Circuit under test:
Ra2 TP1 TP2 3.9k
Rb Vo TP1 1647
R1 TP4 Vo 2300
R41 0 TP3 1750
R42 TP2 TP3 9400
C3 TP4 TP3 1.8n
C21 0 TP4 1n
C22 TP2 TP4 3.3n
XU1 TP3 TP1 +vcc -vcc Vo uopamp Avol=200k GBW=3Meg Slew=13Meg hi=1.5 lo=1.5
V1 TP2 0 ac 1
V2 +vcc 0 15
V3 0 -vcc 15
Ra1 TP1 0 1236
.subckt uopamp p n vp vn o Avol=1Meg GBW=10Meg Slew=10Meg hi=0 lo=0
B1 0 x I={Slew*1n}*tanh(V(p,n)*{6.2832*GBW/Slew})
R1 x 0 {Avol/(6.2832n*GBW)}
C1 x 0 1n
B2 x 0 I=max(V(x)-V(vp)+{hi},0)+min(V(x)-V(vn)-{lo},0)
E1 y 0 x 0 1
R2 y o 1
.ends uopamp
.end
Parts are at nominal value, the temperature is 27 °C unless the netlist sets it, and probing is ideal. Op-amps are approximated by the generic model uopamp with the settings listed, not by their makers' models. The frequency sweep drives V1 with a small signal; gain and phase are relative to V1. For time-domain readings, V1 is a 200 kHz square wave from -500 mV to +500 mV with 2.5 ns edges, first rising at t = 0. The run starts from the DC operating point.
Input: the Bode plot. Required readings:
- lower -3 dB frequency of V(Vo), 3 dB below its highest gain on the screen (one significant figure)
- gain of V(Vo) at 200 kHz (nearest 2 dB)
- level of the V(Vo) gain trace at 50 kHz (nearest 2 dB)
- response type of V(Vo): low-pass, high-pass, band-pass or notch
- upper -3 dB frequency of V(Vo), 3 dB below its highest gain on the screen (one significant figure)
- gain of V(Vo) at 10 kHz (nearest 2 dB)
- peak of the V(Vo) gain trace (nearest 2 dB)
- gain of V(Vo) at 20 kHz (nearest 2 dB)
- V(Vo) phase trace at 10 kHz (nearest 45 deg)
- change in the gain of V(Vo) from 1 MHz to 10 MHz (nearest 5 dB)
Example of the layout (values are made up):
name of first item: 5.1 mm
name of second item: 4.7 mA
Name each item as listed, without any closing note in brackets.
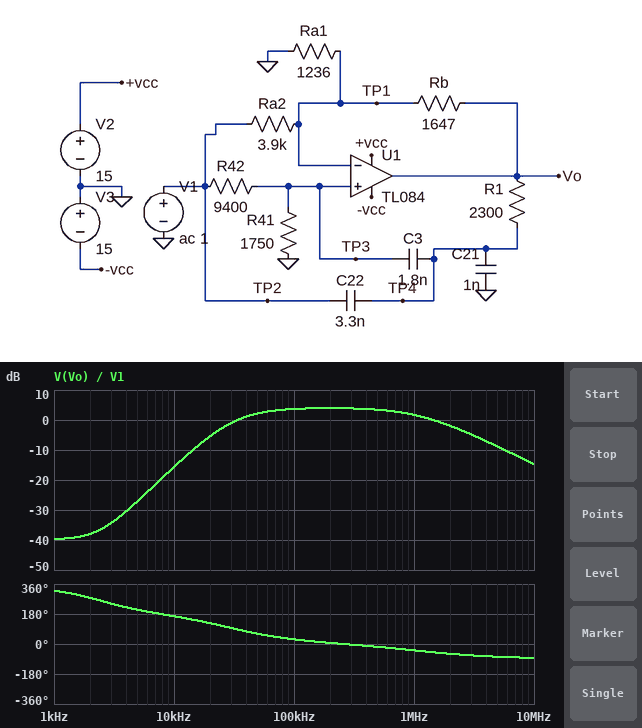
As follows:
lower -3 dB frequency of V(Vo), 3 dB below its highest gain on the screen: 40 kHz
gain of V(Vo) at 200 kHz: 4 dB
level of the V(Vo) gain trace at 50 kHz: 2 dB
response type of V(Vo): low-pass, high-pass, band-pass or notch: band-pass
upper -3 dB frequency of V(Vo), 3 dB below its highest gain on the screen: 1 MHz
gain of V(Vo) at 10 kHz: -16 dB
peak of the V(Vo) gain trace: 4 dB
gain of V(Vo) at 20 kHz: -6 dB
V(Vo) phase trace at 10 kHz: 180 deg
change in the gain of V(Vo) from 1 MHz to 10 MHz: -15 dB
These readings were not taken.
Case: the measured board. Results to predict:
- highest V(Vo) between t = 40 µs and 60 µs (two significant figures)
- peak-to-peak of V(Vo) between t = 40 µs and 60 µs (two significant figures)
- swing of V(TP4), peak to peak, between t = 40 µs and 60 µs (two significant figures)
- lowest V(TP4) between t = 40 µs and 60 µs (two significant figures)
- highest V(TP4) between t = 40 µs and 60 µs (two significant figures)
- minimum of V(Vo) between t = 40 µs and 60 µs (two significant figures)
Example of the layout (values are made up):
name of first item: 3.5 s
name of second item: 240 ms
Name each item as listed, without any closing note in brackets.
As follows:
highest V(Vo) between t = 40 µs and 60 µs: 980 mV
peak-to-peak of V(Vo) between t = 40 µs and 60 µs: 2.0 V
swing of V(TP4), peak to peak, between t = 40 µs and 60 µs: 790 mV
lowest V(TP4) between t = 40 µs and 60 µs: -400 mV
highest V(TP4) between t = 40 µs and 60 µs: 400 mV
minimum of V(Vo) between t = 40 µs and 60 µs: -980 mV
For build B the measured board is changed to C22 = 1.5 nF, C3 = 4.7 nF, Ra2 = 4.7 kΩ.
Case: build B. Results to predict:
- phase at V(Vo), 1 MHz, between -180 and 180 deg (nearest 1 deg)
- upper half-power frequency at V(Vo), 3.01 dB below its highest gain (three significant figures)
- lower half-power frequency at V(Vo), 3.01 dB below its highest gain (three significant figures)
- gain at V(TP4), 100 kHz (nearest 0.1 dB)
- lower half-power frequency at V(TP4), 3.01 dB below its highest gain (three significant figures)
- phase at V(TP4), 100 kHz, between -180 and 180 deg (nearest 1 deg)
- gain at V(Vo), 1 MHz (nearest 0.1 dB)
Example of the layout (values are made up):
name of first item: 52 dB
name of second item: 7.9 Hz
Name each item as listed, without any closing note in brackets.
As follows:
phase at V(Vo), 1 MHz, between -180 and 180 deg: -39 deg
upper half-power frequency at V(Vo), 3.01 dB below its highest gain: 261 kHz
lower half-power frequency at V(Vo), 3.01 dB below its highest gain: 20.8 kHz
gain at V(TP4), 100 kHz: -4.4 dB
lower half-power frequency at V(TP4), 3.01 dB below its highest gain: 19.6 kHz
phase at V(TP4), 100 kHz, between -180 and 180 deg: 1 deg
gain at V(Vo), 1 MHz: -0.9 dB
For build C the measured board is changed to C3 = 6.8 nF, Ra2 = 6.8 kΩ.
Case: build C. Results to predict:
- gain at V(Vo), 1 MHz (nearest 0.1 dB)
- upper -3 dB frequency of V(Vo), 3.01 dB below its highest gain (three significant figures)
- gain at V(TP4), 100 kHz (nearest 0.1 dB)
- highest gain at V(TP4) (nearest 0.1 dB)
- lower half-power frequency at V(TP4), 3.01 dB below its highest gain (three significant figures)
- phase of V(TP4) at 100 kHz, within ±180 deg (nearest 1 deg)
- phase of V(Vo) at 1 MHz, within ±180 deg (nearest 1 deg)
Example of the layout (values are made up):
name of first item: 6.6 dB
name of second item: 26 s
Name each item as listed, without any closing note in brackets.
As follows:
gain at V(Vo), 1 MHz: 2.2 dB
upper -3 dB frequency of V(Vo), 3.01 dB below its highest gain: 903 kHz
gain at V(TP4), 100 kHz: -2.4 dB
highest gain at V(TP4): 0.3 dB
lower half-power frequency at V(TP4), 3.01 dB below its highest gain: 11.8 kHz
phase of V(TP4) at 100 kHz, within ±180 deg: 0 deg
phase of V(Vo) at 1 MHz, within ±180 deg: -39 deg
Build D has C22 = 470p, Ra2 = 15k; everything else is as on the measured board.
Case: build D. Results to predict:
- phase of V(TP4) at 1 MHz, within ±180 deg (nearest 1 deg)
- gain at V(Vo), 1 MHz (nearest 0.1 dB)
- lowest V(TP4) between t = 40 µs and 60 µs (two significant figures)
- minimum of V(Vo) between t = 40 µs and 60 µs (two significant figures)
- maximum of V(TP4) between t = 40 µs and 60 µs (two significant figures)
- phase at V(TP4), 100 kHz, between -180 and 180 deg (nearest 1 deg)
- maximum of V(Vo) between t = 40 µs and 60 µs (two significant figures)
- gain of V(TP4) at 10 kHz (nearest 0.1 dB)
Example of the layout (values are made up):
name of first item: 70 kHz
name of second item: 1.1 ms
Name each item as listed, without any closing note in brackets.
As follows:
phase of V(TP4) at 1 MHz, within ±180 deg: 1 deg
gain at V(Vo), 1 MHz: -6.2 dB
lowest V(TP4) between t = 40 µs and 60 µs: -170 mV
minimum of V(Vo) between t = 40 µs and 60 µs: -330 mV
maximum of V(TP4) between t = 40 µs and 60 µs: 170 mV
phase at V(TP4), 100 kHz, between -180 and 180 deg: -6 deg
maximum of V(Vo) between t = 40 µs and 60 µs: 330 mV
gain of V(TP4) at 10 kHz: -11.1 dB
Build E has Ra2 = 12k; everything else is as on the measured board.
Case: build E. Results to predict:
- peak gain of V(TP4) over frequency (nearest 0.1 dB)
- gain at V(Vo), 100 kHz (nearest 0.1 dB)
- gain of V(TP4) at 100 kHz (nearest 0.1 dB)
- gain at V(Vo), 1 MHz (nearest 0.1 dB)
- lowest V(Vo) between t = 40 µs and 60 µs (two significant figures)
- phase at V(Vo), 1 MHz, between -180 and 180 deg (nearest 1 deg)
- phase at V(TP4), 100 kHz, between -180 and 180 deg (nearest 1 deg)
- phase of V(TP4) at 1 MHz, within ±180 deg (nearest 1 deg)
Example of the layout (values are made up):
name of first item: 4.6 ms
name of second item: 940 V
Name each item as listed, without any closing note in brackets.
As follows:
peak gain of V(TP4) over frequency: -1.5 dB
gain at V(Vo), 100 kHz: 3.8 dB
gain of V(TP4) at 100 kHz: -2.1 dB
gain at V(Vo), 1 MHz: 2.5 dB
lowest V(Vo) between t = 40 µs and 60 µs: -1.0 V
phase at V(Vo), 1 MHz, between -180 and 180 deg: -36 deg
phase at V(TP4), 100 kHz, between -180 and 180 deg: 1 deg
phase of V(TP4) at 1 MHz, within ±180 deg: 1 deg
